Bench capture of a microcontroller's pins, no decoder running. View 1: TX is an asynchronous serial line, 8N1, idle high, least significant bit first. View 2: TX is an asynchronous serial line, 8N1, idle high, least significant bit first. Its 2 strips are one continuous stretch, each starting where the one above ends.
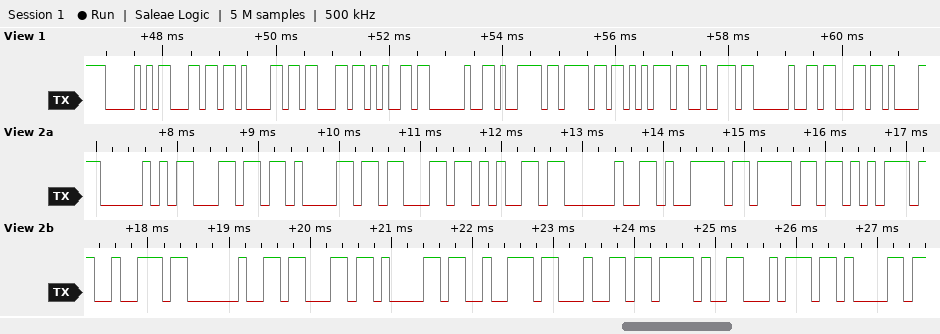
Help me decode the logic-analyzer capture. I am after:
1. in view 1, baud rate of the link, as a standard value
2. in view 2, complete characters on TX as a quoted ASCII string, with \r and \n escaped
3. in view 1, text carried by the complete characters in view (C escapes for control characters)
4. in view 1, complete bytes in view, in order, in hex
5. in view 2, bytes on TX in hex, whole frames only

9600 baud
"Place your card/ta"
"Place your c"
0x50 0x6C 0x61 0x63 0x65 0x20 0x79 0x6F 0x75 0x72 0x20 0x63
50 6C 61 63 65 20 79 6F 75 72 20 63 61 72 64 2F 74 61
